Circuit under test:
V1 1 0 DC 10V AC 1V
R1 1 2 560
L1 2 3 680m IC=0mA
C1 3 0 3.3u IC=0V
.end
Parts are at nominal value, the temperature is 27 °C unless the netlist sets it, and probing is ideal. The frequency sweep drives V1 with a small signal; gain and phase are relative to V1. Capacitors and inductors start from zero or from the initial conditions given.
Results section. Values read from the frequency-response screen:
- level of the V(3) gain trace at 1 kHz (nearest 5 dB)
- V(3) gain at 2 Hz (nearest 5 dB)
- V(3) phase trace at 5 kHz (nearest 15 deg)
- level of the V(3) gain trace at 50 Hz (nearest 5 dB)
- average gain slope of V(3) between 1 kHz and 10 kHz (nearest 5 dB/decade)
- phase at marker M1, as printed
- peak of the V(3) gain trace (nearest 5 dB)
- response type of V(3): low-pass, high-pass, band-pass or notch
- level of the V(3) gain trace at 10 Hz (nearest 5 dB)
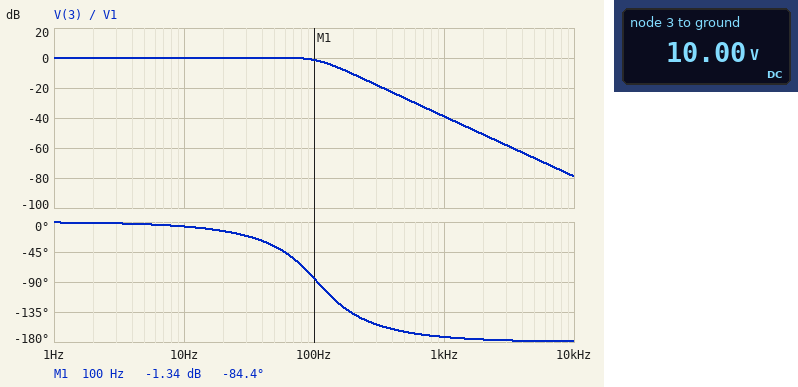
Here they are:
-40 dB
0 dB
-180 deg
0 dB
-40 dB/decade
-84.4 deg
0 dB
low-pass
0 dB
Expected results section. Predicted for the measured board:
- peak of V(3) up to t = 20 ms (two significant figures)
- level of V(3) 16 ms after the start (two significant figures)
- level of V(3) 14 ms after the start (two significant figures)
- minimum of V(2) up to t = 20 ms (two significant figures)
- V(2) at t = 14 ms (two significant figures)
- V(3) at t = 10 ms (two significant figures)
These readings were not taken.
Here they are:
11 V
10 V
10 V
3.9 V
10 V
10 V
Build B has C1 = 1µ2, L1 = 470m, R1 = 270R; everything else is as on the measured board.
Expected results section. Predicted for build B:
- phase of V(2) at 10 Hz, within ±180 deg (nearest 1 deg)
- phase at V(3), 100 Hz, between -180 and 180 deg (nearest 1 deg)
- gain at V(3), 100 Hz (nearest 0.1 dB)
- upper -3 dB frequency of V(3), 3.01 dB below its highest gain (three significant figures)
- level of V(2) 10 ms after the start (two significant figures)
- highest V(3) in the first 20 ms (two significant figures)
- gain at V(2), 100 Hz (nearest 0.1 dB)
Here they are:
-1 deg
-15 deg
1.9 dB
244 Hz
9.9 V
15 V
-0.3 dB
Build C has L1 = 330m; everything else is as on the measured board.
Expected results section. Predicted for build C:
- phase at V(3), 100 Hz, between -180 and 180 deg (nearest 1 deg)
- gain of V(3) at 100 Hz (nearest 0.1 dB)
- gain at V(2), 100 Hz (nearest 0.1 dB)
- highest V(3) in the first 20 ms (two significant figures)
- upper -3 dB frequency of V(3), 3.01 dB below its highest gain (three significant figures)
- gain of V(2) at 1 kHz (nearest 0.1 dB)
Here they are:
-64 deg
-2.2 dB
-7.1 dB
10 V
116 Hz
-0.3 dB
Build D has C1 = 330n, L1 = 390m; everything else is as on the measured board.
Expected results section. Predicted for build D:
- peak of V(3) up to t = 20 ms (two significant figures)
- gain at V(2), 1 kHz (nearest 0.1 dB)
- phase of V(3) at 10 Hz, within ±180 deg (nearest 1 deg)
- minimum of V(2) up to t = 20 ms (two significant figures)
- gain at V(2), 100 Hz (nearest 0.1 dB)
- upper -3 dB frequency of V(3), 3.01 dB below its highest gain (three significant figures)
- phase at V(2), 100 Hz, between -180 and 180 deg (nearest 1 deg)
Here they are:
14 V
-0.3 dB
-1 deg
6.4 V
-0.1 dB
518 Hz
-7 deg
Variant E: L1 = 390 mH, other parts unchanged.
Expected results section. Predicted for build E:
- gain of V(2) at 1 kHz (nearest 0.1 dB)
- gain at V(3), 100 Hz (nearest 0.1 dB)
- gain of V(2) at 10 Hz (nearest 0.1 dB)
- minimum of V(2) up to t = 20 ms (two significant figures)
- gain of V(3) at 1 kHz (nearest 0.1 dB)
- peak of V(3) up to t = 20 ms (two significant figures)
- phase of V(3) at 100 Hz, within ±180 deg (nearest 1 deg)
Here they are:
-0.2 dB
-2.0 dB
-0.1 dB
3.2 V
-34.2 dB
10 V
-67 deg
